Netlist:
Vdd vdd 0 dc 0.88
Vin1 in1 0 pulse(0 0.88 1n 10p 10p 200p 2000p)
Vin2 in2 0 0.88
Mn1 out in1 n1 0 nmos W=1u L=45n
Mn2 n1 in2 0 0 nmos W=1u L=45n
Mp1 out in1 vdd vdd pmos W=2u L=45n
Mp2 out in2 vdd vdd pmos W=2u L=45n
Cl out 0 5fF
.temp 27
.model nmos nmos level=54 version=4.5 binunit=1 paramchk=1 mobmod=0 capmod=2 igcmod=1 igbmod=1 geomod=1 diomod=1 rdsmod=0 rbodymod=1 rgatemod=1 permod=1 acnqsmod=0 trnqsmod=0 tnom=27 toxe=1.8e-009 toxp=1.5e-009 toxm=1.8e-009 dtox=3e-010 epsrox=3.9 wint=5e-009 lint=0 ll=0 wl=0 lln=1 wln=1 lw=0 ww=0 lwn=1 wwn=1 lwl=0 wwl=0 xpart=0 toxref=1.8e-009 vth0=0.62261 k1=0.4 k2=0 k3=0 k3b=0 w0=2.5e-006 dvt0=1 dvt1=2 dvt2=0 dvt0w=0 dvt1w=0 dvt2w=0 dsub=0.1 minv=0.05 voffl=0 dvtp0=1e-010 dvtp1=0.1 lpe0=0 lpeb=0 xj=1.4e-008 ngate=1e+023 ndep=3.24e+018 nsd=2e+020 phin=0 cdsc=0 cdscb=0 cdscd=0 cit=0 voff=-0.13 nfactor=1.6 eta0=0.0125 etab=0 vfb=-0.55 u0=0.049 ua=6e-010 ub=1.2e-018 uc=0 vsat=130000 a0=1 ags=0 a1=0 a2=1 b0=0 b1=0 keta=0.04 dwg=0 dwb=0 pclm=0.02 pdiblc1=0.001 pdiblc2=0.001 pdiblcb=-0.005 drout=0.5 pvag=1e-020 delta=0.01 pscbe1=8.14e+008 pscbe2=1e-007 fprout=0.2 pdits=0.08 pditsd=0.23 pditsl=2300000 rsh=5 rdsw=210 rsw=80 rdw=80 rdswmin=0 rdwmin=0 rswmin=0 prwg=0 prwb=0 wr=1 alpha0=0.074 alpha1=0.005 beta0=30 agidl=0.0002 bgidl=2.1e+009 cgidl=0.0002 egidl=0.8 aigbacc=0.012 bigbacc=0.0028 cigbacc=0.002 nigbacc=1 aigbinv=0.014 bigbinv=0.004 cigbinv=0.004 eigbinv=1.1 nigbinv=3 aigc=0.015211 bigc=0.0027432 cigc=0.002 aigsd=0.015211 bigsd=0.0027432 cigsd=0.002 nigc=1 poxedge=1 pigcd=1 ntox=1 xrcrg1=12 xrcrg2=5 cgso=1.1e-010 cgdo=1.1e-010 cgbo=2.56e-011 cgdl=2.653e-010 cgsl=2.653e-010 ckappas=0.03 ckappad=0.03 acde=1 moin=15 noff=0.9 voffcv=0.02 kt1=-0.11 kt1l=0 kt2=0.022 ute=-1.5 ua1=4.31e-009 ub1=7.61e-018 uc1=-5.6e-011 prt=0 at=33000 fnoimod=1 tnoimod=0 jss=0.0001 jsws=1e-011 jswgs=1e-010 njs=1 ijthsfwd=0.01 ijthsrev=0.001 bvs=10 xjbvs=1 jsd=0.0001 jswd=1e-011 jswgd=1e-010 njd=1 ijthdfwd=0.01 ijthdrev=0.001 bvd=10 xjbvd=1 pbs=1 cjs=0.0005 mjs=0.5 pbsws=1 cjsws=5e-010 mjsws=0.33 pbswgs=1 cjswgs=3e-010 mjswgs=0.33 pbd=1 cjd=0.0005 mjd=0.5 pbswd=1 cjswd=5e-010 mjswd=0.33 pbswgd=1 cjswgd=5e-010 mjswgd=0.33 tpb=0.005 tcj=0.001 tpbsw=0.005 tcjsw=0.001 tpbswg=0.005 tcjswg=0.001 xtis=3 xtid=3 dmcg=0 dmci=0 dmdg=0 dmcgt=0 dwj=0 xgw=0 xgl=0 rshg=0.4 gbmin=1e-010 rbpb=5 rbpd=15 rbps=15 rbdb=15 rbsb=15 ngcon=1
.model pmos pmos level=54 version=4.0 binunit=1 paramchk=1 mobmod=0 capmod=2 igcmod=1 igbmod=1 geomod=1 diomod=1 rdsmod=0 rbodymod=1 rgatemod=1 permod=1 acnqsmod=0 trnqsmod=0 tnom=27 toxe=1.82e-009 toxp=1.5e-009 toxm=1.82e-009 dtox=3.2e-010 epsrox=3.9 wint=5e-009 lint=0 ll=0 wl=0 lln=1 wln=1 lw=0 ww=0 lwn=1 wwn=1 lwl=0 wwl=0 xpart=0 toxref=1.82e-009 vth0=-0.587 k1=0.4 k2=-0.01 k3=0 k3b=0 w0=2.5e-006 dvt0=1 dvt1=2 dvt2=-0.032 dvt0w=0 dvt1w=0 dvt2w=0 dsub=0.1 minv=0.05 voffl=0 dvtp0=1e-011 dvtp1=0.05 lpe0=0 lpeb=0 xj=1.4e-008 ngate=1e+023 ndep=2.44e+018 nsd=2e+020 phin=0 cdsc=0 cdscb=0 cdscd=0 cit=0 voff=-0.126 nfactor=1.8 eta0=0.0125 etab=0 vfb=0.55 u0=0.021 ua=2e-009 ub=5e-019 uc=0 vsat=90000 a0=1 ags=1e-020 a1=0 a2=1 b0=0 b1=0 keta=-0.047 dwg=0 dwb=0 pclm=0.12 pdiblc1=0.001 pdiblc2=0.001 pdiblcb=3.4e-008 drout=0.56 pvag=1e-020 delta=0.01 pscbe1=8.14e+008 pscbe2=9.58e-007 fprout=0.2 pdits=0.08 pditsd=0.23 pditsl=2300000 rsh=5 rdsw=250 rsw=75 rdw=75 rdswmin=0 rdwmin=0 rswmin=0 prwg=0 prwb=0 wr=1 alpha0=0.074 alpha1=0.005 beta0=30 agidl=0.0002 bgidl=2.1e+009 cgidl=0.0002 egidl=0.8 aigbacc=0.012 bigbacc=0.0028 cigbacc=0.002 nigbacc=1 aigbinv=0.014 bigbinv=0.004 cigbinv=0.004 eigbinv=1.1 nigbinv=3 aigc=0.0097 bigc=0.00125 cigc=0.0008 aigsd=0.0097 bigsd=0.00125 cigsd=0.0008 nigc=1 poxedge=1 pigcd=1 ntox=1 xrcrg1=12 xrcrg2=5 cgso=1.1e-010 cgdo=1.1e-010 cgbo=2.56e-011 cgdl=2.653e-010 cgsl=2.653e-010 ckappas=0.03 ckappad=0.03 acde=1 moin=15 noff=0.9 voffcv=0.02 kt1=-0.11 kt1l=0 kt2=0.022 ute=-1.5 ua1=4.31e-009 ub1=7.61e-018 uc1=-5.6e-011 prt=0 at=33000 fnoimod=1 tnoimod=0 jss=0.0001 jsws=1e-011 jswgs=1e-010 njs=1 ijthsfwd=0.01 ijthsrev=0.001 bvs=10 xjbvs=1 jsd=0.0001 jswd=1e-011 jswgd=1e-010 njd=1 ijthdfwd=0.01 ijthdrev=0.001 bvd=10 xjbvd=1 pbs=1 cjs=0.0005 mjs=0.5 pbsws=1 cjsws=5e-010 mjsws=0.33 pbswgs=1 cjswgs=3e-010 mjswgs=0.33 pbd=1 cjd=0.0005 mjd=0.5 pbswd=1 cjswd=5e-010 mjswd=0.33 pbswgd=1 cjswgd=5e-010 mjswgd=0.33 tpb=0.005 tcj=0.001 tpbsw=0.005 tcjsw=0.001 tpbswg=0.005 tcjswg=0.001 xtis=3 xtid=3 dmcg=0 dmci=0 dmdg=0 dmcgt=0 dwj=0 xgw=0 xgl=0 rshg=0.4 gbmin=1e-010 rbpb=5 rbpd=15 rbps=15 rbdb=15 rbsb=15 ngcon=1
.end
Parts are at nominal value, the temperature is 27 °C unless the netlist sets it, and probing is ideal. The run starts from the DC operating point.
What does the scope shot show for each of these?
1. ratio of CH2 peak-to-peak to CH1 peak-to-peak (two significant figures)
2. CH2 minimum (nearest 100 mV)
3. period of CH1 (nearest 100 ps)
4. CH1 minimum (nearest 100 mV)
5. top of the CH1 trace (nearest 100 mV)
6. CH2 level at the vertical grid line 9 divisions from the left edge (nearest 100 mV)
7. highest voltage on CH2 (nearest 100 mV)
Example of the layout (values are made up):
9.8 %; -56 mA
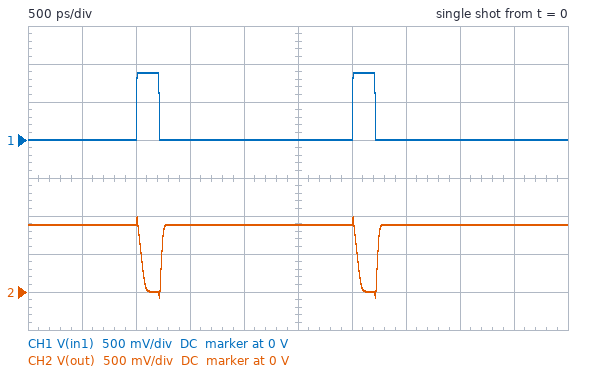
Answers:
1.2; -100 mV; 2.0 ns; 0 V; 900 mV; 900 mV; 1.0 V
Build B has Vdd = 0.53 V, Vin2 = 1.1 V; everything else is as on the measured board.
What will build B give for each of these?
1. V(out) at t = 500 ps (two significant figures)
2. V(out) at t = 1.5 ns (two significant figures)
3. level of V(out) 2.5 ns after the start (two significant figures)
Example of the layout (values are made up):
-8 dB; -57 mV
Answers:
530 mV; 94 mV; 500 mV
